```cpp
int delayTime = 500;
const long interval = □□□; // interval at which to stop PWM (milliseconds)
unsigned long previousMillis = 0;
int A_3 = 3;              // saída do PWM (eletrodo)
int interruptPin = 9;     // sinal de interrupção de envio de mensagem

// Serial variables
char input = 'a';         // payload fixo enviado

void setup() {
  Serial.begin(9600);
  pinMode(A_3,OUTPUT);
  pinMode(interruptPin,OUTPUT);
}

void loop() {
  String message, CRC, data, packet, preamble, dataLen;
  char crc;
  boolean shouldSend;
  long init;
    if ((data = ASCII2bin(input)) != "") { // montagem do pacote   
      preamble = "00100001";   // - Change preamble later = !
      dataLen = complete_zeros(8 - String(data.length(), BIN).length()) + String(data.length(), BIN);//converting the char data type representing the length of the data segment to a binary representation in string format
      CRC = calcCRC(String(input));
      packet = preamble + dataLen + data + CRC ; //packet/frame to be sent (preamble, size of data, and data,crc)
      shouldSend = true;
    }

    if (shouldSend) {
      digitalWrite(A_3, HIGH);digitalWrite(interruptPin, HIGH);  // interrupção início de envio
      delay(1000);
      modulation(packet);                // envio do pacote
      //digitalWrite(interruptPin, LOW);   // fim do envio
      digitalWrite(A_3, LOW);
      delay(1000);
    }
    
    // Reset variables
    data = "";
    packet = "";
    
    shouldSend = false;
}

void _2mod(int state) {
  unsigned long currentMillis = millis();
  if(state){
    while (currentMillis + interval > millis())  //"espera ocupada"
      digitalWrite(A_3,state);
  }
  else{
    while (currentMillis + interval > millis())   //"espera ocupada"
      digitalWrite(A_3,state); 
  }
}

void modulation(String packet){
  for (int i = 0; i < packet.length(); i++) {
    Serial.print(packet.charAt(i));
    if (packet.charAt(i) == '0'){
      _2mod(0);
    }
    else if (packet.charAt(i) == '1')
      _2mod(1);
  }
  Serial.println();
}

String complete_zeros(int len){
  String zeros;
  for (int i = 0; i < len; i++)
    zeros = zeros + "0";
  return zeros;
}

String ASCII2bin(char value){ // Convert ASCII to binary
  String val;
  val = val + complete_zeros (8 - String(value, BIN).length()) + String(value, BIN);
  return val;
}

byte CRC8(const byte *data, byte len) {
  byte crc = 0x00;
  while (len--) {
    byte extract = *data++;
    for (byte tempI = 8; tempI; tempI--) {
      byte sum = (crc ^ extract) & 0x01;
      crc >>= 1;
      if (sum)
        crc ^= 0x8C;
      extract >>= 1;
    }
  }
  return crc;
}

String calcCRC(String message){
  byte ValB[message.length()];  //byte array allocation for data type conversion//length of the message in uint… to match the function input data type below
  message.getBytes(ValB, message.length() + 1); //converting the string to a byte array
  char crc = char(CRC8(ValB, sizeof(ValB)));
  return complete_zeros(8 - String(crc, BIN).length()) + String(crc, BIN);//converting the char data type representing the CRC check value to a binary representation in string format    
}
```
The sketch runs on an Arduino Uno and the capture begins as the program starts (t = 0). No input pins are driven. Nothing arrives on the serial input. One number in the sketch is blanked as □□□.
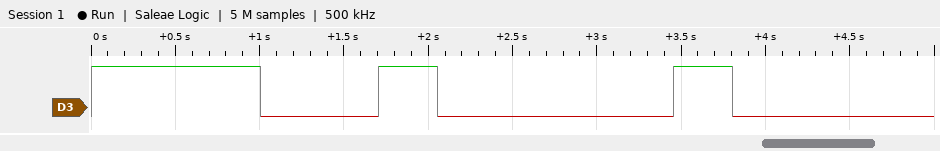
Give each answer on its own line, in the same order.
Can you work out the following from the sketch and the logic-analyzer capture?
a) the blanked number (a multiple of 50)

350
